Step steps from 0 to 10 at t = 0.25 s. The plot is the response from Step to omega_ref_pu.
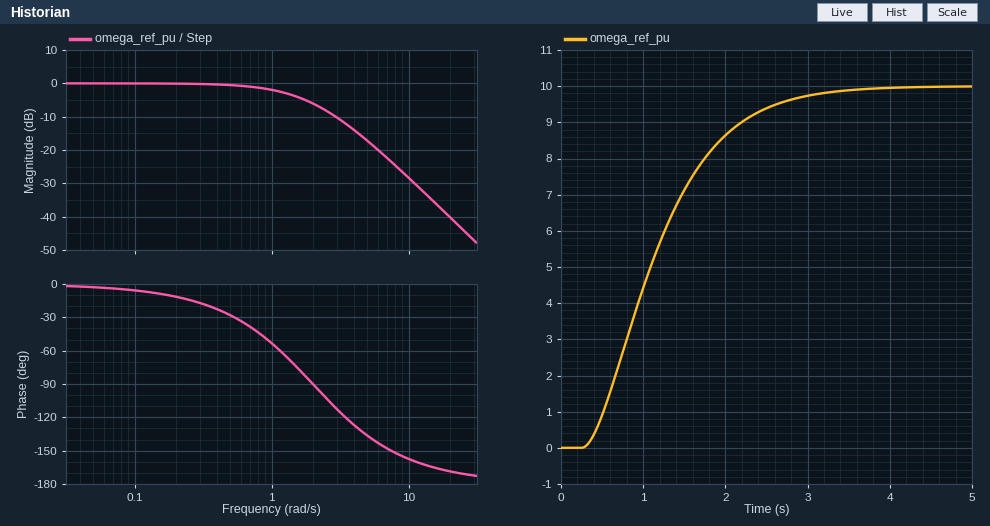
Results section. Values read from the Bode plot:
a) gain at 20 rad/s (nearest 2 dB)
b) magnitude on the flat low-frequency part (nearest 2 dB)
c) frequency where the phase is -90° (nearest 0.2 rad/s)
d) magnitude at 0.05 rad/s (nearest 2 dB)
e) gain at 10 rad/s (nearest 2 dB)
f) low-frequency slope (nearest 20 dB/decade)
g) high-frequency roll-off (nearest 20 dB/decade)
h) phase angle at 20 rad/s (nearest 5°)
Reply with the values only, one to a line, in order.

-40 dB
0 dB
2.0 rad/s
0 dB
-28 dB
0 dB/decade
-40 dB/decade
-170°
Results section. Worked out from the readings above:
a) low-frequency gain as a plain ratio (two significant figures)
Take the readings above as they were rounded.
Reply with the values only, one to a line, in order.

1.0
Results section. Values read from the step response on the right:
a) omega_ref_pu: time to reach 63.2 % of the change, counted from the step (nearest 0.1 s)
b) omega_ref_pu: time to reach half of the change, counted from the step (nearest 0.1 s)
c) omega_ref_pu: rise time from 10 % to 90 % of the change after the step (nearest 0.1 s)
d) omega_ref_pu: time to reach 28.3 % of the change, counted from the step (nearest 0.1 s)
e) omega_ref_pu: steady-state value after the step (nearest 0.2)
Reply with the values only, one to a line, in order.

1.1 s
0.8 s
1.7 s
0.5 s
10.0
